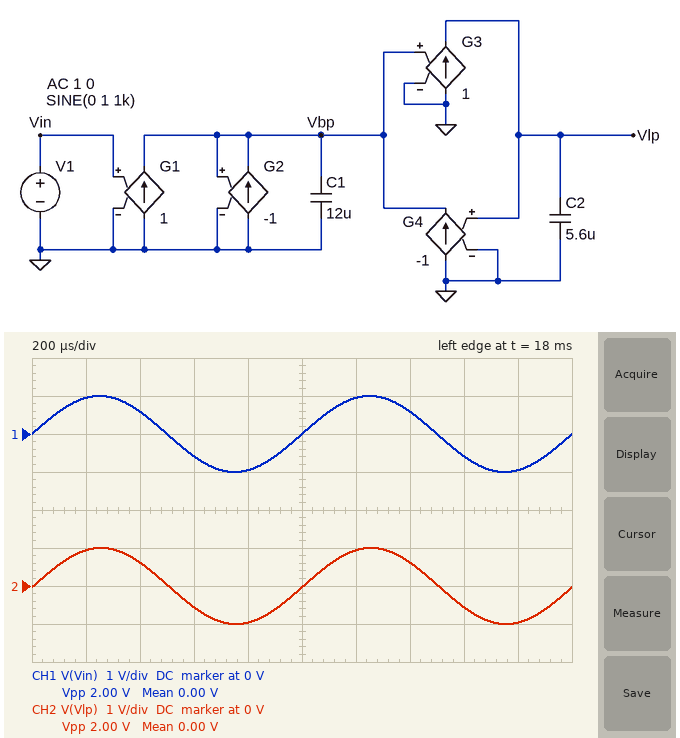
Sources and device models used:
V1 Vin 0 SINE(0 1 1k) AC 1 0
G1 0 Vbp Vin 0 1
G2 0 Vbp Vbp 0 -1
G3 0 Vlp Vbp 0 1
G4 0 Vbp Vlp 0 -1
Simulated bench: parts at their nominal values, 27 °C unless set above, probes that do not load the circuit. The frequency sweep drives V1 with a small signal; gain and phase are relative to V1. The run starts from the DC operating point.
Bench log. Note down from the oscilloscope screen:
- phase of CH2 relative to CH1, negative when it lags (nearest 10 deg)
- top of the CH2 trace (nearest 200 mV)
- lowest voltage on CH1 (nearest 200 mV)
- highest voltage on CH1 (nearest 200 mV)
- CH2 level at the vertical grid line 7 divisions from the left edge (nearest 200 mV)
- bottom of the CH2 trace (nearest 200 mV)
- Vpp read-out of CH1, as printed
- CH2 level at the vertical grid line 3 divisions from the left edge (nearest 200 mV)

0 deg
1.0 V
-1.0 V
1.0 V
600 mV
-1.0 V
2.00 V
-600 mV
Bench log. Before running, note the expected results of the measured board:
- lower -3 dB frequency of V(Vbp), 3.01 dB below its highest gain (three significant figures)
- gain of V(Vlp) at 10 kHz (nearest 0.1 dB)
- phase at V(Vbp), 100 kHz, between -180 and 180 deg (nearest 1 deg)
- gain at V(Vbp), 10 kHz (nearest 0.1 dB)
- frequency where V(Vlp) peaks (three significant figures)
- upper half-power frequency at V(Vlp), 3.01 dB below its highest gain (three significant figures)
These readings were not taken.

13.9 kHz
1.8 dB
-82 deg
-7.3 dB
17.0 kHz
23.0 kHz
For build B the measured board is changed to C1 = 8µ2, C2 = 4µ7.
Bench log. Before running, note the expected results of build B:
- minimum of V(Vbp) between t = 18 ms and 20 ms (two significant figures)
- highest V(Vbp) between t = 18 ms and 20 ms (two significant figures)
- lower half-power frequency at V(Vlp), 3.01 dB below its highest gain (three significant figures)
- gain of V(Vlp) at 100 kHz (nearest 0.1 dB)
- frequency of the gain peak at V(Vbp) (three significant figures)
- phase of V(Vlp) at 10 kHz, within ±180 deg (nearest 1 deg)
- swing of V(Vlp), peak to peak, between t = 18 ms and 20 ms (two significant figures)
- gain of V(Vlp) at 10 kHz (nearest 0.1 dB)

-30 mV
30 mV
2.89 kHz
-23.2 dB
25.6 kHz
-19 deg
2.0 V
0.9 dB
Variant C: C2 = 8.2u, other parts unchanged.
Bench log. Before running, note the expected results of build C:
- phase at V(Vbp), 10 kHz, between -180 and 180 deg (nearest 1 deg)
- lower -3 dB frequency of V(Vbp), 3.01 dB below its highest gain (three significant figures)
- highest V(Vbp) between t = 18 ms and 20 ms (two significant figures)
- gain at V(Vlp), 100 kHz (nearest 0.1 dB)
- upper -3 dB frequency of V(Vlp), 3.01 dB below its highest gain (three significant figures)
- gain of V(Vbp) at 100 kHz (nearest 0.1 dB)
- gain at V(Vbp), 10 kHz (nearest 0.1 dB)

50 deg
10.7 kHz
52 mV
-31.6 dB
19.1 kHz
-17.4 dB
-3.8 dB
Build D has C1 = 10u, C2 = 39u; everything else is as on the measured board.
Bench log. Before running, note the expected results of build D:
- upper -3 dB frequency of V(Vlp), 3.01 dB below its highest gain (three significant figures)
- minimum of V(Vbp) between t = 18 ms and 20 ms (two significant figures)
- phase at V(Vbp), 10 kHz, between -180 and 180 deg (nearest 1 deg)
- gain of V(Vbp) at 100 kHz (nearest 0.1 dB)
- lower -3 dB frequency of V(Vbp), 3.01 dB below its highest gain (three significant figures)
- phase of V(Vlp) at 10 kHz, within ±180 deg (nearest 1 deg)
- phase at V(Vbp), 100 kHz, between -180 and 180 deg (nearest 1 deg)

5.28 kHz
-240 mV
-12 deg
-16.0 dB
3.37 kHz
-102 deg
-81 deg
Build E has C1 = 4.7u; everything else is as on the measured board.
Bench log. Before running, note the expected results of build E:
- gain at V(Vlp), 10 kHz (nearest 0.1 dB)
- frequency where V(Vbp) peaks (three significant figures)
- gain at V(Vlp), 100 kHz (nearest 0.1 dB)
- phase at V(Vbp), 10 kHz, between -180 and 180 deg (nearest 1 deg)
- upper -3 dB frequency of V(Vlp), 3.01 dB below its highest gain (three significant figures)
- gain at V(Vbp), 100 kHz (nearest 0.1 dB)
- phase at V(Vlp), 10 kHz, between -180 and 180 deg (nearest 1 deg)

0.3 dB
31.0 kHz
-20.0 dB
69 deg
35.6 kHz
-9.1 dB
-21 deg
